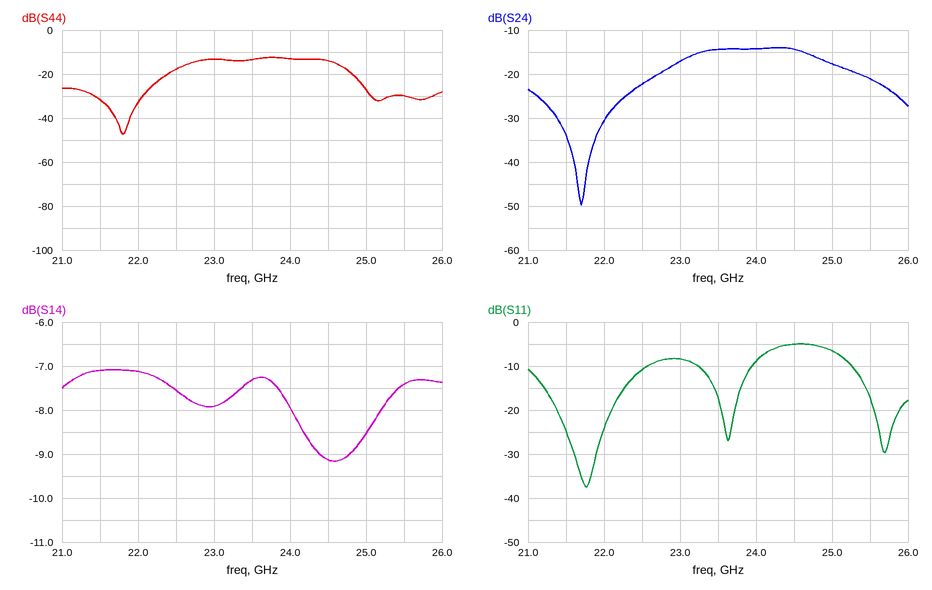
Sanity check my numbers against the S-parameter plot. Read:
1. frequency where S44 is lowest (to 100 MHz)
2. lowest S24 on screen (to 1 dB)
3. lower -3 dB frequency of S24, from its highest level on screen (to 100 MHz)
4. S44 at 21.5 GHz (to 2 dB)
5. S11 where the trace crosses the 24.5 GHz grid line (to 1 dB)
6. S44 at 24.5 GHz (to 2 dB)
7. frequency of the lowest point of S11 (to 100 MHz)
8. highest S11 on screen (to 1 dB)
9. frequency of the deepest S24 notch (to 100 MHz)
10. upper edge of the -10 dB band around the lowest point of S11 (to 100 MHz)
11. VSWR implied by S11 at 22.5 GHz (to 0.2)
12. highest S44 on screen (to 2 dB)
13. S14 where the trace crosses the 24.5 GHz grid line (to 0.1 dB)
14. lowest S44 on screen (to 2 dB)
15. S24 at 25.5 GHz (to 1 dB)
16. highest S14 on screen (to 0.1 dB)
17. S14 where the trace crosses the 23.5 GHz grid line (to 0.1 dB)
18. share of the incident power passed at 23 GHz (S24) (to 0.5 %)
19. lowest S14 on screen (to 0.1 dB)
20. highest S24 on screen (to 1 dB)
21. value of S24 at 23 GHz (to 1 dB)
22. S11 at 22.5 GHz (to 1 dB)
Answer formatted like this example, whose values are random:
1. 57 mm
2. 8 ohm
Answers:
1. 21.8 GHz
2. -50 dB
3. 23.0 GHz
4. -32 dB
5. -5 dB
6. -14 dB
7. 21.8 GHz
8. -5 dB
9. 21.7 GHz
10. 22.6 GHz
11. 1.8
12. -12 dB
13. -9.1 dB
14. -48 dB
15. -21 dB
16. -7.1 dB
17. -7.3 dB
18. 2.0 %
19. -9.2 dB
20. -14 dB
21. -17 dB
22. -11 dB
